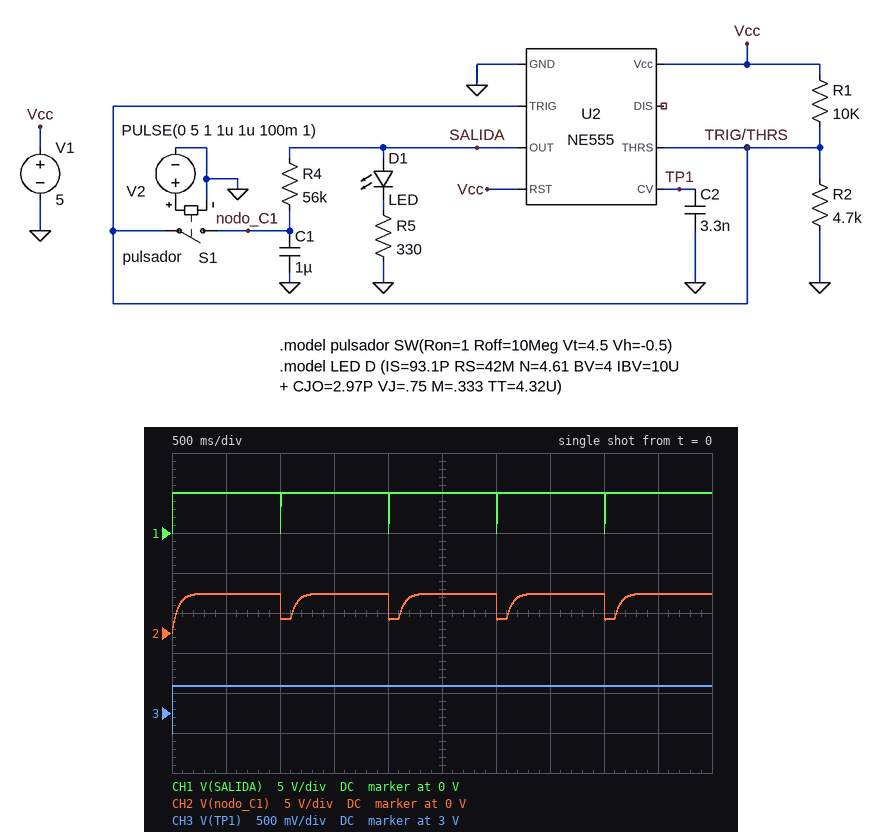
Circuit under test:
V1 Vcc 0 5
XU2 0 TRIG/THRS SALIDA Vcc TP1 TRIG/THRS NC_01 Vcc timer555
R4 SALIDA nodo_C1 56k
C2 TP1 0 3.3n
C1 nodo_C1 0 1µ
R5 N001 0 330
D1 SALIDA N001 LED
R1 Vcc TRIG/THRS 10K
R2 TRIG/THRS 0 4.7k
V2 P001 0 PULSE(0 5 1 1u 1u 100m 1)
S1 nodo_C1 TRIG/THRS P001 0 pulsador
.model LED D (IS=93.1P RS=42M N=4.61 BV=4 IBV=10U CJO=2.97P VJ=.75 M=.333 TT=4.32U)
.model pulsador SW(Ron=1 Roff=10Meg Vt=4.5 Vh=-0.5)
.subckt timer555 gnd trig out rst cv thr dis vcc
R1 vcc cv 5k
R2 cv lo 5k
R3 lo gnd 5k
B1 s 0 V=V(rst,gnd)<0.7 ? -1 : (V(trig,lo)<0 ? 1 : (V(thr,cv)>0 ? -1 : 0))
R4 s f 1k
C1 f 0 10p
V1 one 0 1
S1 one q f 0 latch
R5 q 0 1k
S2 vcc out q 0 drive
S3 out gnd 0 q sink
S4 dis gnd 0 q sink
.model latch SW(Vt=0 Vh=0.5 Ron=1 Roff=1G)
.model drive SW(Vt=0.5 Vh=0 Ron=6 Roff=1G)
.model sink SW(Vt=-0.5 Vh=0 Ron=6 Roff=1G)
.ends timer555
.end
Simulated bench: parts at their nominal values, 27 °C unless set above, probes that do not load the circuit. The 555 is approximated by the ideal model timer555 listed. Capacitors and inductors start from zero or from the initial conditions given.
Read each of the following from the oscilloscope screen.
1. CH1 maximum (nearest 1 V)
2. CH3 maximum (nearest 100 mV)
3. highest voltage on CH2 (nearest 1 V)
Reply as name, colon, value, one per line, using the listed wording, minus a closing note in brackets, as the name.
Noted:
CH1 maximum: 5 V
CH3 maximum: 3.3 V
highest voltage on CH2: 5 V
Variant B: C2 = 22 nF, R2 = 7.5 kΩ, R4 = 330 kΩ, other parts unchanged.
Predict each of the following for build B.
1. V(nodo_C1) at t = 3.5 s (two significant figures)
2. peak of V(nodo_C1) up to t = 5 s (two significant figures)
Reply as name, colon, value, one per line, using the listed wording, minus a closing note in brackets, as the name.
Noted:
V(nodo_C1) at t = 3.5 s: 4.1 V
peak of V(nodo_C1) up to t = 5 s: 4.7 V
